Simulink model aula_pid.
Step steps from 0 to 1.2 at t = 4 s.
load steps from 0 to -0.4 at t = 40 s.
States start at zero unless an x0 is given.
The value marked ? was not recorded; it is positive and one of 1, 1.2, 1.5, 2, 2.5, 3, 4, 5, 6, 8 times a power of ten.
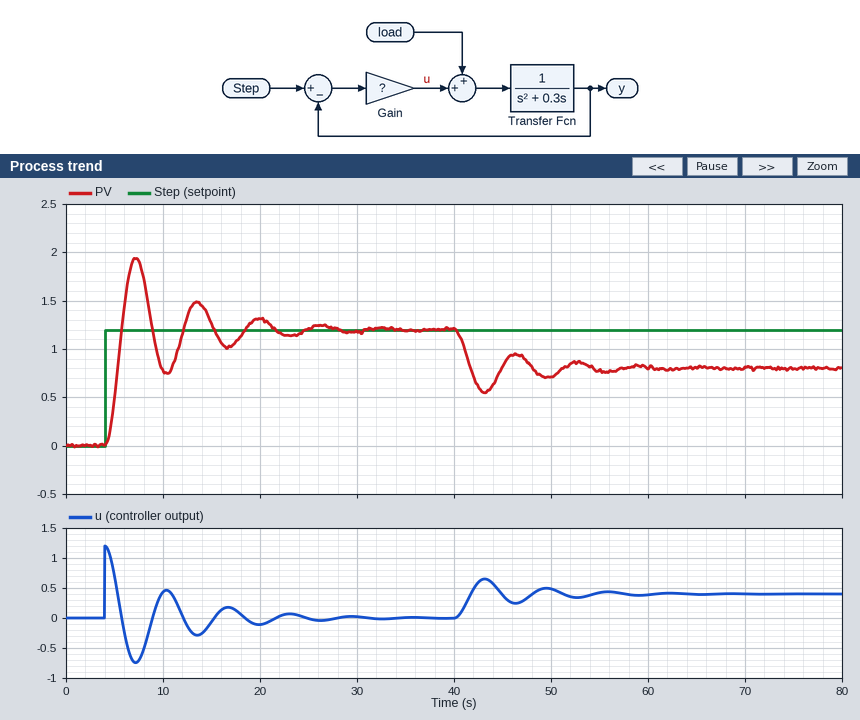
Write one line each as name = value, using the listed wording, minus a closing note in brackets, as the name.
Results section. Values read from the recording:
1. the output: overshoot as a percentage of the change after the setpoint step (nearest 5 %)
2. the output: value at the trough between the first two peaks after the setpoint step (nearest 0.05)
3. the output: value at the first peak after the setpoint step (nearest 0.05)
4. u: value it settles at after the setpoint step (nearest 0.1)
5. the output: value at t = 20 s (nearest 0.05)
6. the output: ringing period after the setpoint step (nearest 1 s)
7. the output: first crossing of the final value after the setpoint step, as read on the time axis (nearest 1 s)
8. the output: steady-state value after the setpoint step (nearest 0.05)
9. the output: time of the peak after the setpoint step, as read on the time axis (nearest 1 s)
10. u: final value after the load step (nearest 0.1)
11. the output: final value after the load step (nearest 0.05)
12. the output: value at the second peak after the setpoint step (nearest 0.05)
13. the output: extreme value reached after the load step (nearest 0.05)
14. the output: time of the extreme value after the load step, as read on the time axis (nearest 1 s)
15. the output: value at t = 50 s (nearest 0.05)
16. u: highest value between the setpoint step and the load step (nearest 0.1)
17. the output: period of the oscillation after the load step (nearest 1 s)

the output: overshoot as a percentage of the change after the setpoint step = 60 %
the output: value at the trough between the first two peaks after the setpoint step = 0.75
the output: value at the first peak after the setpoint step = 1.95
u: value it settles at after the setpoint step = 0.0
the output: value at t = 20 s = 1.30
the output: ringing period after the setpoint step = 6 s
the output: first crossing of the final value after the setpoint step, as read on the time axis = 6 s
the output: steady-state value after the setpoint step = 1.20
the output: time of the peak after the setpoint step, as read on the time axis = 7 s
u: final value after the load step = 0.4
the output: final value after the load step = 0.80
the output: value at the second peak after the setpoint step = 1.50
the output: extreme value reached after the load step = 0.55
the output: time of the extreme value after the load step, as read on the time axis = 43 s
the output: value at t = 50 s = 0.70
u: highest value between the setpoint step and the load step = 1.2
the output: period of the oscillation after the load step = 6 s
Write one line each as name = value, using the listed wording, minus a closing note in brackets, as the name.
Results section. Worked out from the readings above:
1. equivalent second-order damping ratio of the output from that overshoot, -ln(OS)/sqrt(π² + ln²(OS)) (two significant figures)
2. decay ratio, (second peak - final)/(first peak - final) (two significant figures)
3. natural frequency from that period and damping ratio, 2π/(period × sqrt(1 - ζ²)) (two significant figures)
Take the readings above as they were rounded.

equivalent second-order damping ratio of the output from that overshoot, -ln(OS)/sqrt(π² + ln²(OS)) = 0.16
decay ratio, (second peak - final)/(first peak - final) = 0.40
natural frequency from that period and damping ratio, 2π/(period × sqrt(1 - ζ²)) = 1.1 rad/s
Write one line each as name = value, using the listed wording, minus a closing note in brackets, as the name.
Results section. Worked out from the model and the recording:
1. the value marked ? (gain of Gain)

the value marked ? = 1
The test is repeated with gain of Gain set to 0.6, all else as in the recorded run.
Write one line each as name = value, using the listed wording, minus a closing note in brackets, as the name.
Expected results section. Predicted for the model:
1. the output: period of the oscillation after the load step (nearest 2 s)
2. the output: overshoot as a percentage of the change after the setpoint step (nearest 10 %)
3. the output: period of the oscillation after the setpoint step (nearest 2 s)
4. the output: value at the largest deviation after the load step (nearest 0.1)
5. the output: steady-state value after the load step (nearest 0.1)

the output: period of the oscillation after the load step = 8 s
the output: overshoot as a percentage of the change after the setpoint step = 50 %
the output: period of the oscillation after the setpoint step = 8 s
the output: value at the largest deviation after the load step = 0.2
the output: steady-state value after the load step = 0.5
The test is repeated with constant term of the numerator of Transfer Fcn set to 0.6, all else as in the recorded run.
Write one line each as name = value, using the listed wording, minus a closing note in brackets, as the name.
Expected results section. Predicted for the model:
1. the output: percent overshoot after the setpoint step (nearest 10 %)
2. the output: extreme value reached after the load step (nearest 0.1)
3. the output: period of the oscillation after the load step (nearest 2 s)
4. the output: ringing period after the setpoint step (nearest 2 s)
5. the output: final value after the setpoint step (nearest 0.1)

the output: percent overshoot after the setpoint step = 50 %
the output: extreme value reached after the load step = 0.6
the output: period of the oscillation after the load step = 8 s
the output: ringing period after the setpoint step = 8 s
the output: final value after the setpoint step = 1.2
